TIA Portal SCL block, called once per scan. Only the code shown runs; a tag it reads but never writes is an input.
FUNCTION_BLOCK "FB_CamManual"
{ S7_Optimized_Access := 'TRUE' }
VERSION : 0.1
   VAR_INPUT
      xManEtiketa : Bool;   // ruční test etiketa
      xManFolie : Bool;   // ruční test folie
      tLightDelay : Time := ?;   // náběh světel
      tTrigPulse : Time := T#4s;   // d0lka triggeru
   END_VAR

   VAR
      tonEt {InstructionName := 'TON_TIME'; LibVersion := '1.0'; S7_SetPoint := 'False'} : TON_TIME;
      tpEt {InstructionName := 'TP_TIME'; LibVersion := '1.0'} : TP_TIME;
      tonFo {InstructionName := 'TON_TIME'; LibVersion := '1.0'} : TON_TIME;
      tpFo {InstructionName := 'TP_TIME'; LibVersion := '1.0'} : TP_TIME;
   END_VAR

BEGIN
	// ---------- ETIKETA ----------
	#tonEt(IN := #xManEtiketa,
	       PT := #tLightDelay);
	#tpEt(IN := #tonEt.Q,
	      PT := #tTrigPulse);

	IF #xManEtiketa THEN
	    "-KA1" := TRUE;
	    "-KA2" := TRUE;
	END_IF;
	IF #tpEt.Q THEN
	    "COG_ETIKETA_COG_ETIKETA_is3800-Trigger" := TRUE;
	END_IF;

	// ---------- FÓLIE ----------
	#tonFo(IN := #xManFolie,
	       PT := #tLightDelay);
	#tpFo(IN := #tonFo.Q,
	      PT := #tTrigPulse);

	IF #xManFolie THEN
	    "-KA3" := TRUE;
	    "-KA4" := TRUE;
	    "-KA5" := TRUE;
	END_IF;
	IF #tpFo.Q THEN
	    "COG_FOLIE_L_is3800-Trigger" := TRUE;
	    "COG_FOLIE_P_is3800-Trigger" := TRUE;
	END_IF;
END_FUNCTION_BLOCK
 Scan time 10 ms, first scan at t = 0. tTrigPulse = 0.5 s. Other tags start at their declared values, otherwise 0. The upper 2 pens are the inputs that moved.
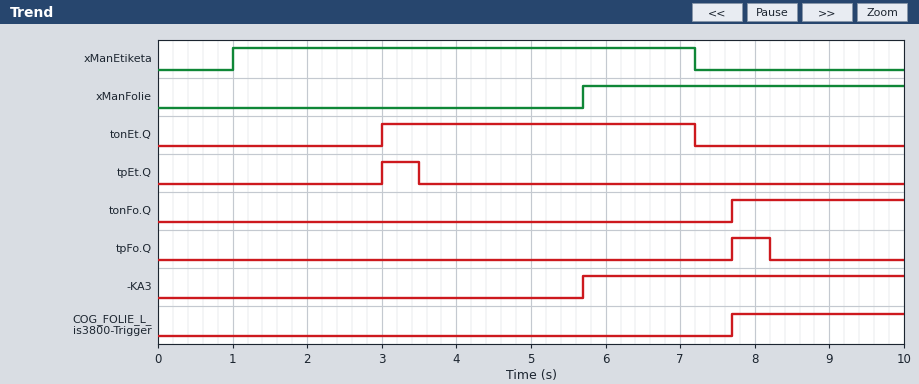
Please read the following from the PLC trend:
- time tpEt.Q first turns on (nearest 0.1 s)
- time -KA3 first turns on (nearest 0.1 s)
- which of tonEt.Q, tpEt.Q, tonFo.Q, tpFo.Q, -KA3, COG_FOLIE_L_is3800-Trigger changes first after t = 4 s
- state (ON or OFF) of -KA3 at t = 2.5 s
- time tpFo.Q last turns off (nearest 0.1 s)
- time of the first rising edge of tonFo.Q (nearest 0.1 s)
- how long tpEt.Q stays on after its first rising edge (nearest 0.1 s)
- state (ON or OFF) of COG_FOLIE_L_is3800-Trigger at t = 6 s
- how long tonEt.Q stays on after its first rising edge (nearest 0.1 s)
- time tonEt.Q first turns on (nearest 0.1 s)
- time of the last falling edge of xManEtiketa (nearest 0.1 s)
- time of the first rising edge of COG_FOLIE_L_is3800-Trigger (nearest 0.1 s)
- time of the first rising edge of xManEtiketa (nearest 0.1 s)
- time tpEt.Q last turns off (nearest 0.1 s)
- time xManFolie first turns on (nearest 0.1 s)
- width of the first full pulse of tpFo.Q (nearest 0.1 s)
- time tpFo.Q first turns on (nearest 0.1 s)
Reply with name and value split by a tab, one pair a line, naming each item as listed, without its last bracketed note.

time tpEt.Q first turns on	3.0 s
time -KA3 first turns on	5.7 s
which of tonEt.Q, tpEt.Q, tonFo.Q, tpFo.Q, -KA3, COG_FOLIE_L_is3800-Trigger changes first after t = 4 s	-KA3
state (ON or OFF) of -KA3 at t = 2.5 s	OFF
time tpFo.Q last turns off	8.2 s
time of the first rising edge of tonFo.Q	7.7 s
how long tpEt.Q stays on after its first rising edge	0.5 s
state (ON or OFF) of COG_FOLIE_L_is3800-Trigger at t = 6 s	OFF
how long tonEt.Q stays on after its first rising edge	4.2 s
time tonEt.Q first turns on	3.0 s
time of the last falling edge of xManEtiketa	7.2 s
time of the first rising edge of COG_FOLIE_L_is3800-Trigger	7.7 s
time of the first rising edge of xManEtiketa	1.0 s
time tpEt.Q last turns off	3.5 s
time xManFolie first turns on	5.7 s
width of the first full pulse of tpFo.Q	0.5 s
time tpFo.Q first turns on	7.7 s
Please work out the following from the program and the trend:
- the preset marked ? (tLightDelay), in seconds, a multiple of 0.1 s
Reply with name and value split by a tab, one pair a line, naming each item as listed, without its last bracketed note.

the preset marked ? (tLightDelay), in seconds, a multiple of 0.1 s	2.0 s
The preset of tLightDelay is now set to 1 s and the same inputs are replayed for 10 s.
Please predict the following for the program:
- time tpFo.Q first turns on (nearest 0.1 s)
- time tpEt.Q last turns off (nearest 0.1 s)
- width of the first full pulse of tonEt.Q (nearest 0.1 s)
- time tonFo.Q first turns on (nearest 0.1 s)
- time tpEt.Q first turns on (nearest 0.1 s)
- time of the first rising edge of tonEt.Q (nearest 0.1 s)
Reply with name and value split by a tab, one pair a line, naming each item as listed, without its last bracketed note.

time tpFo.Q first turns on	6.7 s
time tpEt.Q last turns off	2.5 s
width of the first full pulse of tonEt.Q	5.2 s
time tonFo.Q first turns on	6.7 s
time tpEt.Q first turns on	2.0 s
time of the first rising edge of tonEt.Q	2.0 s
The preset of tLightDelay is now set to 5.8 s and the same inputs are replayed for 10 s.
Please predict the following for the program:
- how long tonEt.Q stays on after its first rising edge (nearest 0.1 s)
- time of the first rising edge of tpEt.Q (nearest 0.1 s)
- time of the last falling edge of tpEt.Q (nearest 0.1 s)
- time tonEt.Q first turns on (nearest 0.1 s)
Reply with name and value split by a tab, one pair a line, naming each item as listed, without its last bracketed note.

how long tonEt.Q stays on after its first rising edge	0.4 s
time of the first rising edge of tpEt.Q	6.8 s
time of the last falling edge of tpEt.Q	7.3 s
time tonEt.Q first turns on	6.8 s
